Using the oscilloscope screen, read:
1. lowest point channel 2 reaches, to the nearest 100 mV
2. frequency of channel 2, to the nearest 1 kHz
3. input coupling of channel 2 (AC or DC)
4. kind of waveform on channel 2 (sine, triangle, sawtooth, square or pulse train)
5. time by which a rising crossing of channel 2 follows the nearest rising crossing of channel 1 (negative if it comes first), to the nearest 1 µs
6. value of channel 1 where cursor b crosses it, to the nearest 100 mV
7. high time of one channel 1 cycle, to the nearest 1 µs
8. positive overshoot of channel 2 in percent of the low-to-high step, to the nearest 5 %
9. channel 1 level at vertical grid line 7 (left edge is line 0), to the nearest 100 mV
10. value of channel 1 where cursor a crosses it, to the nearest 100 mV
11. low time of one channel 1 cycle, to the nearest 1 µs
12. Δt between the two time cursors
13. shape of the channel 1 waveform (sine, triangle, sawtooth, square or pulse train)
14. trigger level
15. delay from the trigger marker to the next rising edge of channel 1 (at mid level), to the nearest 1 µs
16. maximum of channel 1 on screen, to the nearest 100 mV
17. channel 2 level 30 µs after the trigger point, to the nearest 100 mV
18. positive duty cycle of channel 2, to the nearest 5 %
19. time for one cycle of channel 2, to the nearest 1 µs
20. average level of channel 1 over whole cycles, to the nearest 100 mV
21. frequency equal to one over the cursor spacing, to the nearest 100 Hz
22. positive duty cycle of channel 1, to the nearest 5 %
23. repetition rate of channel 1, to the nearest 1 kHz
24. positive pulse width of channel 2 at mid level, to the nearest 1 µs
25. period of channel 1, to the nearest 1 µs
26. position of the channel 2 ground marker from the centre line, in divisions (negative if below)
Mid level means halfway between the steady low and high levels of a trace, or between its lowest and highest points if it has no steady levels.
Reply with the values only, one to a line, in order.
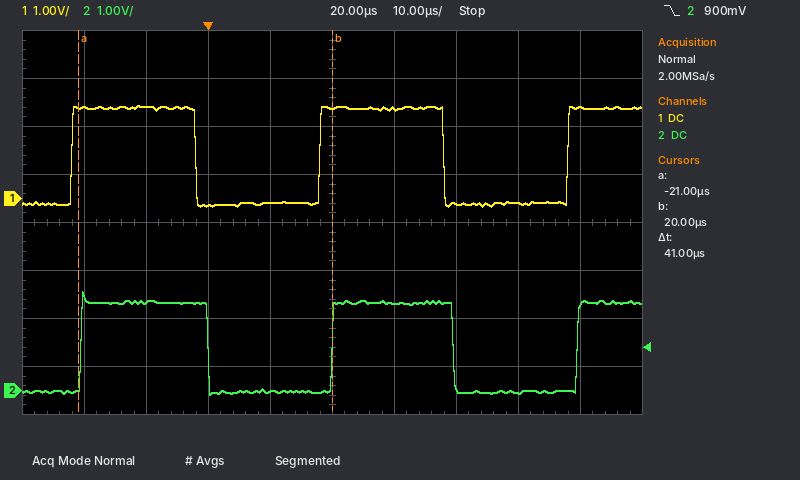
-100 mV
25 kHz
DC
square
+2 µs
1.9 V
20 µs
10 %
-100 mV
1.9 V
20 µs
41 µs
square
900 mV
18 µs
1.9 V
1.8 V
50 %
40 µs
900 mV
24.4 kHz
50 %
25 kHz
20 µs
40 µs
-3.5 div
